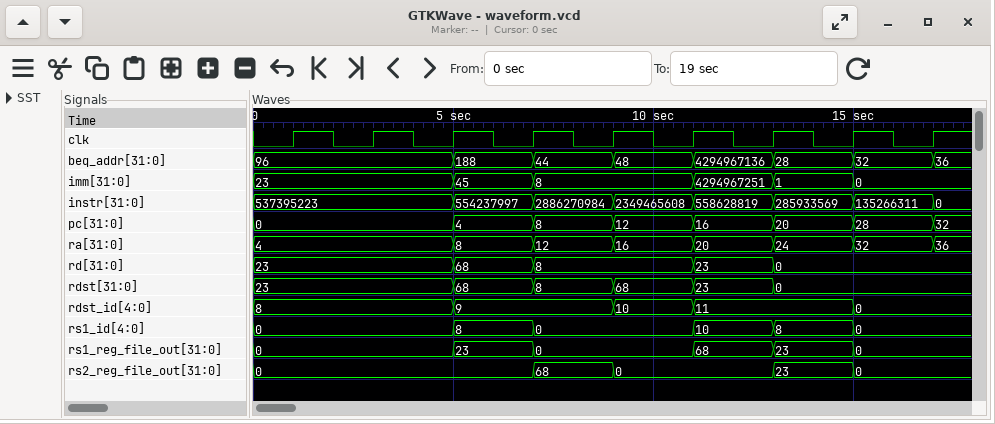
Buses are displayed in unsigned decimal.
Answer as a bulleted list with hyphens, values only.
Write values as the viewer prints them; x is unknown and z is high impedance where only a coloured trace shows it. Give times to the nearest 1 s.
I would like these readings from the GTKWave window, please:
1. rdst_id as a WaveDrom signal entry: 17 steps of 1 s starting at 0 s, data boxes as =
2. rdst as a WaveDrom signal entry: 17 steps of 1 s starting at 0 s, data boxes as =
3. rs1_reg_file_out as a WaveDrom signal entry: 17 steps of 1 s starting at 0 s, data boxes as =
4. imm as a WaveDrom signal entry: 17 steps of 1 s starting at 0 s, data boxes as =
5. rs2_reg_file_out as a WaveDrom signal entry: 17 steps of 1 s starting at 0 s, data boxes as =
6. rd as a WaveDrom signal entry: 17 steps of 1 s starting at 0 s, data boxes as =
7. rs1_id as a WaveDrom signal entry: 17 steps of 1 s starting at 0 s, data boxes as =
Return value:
- {name: 'rdst_id', wave: '=....=...=.=...=.', data: '8 9 10 11 0'}
- {name: 'rdst', wave: '=....=.=.=.=.=...', data: '23 68 8 68 23 0'}
- {name: 'rs1_reg_file_out', wave: '=....=.=...=.=.=.', data: '0 23 0 68 23 0'}
- {name: 'imm', wave: '=....=.=...=.=.=.', data: '23 45 8 4294967251 1 0'}
- {name: 'rs2_reg_file_out', wave: '=......=.=...=.=.', data: '0 68 0 23 0'}
- {name: 'rd', wave: '=....=.=...=.=...', data: '23 68 8 23 0'}
- {name: 'rs1_id', wave: '=....=.=...=.=.=.', data: '0 8 0 10 8 0'}
